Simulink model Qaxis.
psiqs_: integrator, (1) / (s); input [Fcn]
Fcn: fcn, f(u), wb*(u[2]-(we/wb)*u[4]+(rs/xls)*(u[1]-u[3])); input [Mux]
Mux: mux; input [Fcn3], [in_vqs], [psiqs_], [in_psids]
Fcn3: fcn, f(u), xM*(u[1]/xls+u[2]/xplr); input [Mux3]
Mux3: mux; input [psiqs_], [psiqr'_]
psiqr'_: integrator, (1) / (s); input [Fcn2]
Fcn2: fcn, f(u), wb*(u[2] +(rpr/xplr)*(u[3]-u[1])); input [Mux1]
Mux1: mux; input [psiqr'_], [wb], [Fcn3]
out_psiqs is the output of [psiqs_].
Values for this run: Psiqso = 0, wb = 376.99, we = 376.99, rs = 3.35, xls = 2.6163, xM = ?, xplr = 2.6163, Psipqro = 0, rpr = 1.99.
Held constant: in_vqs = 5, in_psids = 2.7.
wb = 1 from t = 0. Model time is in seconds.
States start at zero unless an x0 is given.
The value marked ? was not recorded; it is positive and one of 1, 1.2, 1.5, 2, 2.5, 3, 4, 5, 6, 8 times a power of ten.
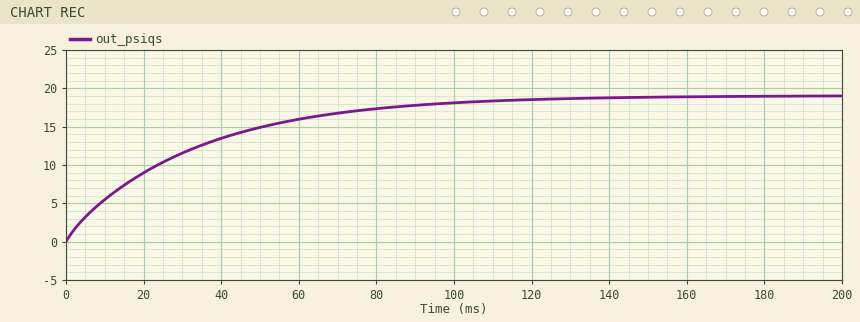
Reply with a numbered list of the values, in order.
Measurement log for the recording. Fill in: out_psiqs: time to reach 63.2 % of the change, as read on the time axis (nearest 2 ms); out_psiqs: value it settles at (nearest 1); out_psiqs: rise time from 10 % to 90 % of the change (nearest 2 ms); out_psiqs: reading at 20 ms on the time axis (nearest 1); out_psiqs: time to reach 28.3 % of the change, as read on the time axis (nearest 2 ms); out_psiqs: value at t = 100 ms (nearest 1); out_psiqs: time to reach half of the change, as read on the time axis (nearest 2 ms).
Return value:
1. 32 ms
2. 19
3. 74 ms
4. 9
5. 10 ms
6. 18
7. 22 ms
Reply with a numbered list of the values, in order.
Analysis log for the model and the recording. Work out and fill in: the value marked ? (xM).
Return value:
1. 1.2
